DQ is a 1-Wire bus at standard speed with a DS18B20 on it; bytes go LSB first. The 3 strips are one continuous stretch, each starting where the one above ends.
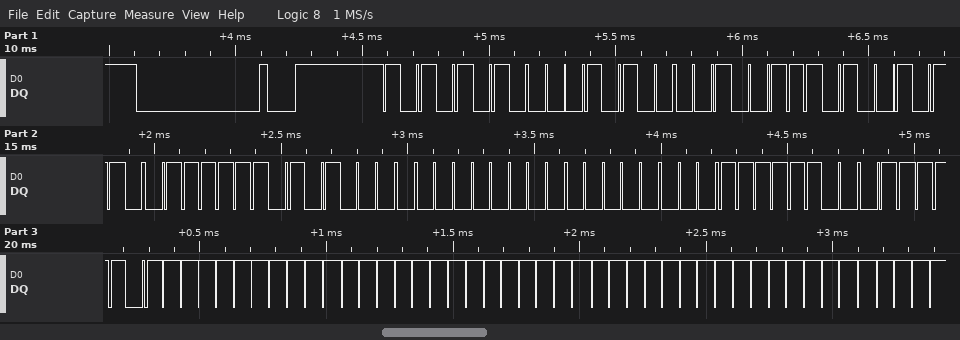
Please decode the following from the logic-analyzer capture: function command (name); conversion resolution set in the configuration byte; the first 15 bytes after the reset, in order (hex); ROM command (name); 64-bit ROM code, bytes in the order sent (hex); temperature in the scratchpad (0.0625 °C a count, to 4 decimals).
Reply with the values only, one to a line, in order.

Read Scratchpad
12 bits
55 28 E4 D2 FC 0A 00 00 3F BE FF FF FF FF FF
Match ROM
28 E4 D2 FC 0A 00 00 3F
-0.0625 °C
